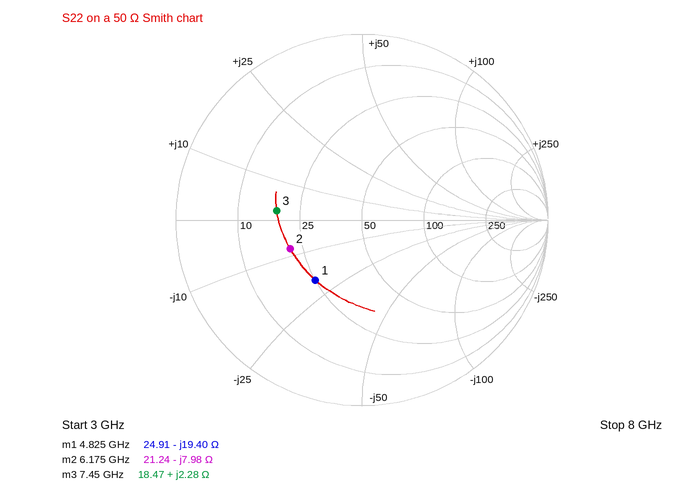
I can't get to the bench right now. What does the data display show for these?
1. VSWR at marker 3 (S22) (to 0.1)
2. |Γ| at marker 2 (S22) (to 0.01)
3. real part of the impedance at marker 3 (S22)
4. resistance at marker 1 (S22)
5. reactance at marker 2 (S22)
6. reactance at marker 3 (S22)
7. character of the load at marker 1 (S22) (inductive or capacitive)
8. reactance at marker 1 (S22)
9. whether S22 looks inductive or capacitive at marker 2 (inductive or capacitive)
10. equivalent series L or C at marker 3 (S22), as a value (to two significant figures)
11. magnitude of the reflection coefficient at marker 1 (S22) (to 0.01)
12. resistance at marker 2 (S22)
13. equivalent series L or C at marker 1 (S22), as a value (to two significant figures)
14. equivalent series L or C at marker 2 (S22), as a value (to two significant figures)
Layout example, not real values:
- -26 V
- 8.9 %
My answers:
- 2.7
- 0.42
- 18.47 Ω
- 24.91 Ω
- -7.98 Ω
- +2.28 Ω
- capacitive
- -19.40 Ω
- capacitive
- 49 pH
- 0.41
- 21.24 Ω
- 1.7 pF
- 3.2 pF
